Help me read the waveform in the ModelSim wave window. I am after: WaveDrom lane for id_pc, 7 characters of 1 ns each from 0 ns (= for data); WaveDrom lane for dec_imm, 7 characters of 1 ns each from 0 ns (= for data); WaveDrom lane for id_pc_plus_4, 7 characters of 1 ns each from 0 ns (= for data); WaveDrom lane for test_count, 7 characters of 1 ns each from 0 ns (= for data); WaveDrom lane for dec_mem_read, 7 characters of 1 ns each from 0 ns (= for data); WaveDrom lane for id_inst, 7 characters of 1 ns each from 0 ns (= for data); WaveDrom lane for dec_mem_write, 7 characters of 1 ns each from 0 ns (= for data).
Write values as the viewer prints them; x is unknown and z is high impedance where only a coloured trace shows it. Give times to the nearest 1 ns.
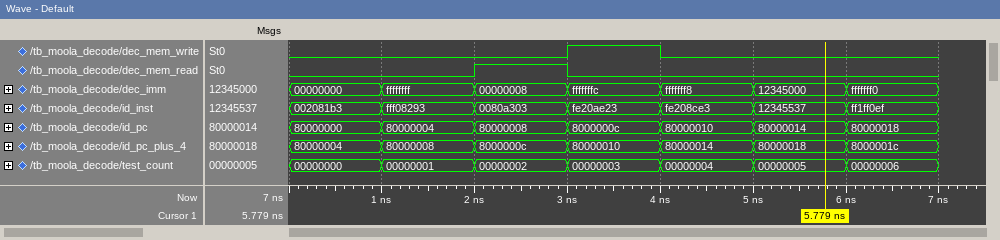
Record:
{name: 'id_pc', wave: '=======', data: '80000000 80000004 80000008 8000000c 80000010 80000014 80000018'}
{name: 'dec_imm', wave: '=======', data: '00000000 ffffffff 00000008 fffffffc fffffff8 12345000 fffffff0'}
{name: 'id_pc_plus_4', wave: '=======', data: '80000004 80000008 8000000c 80000010 80000014 80000018 8000001c'}
{name: 'test_count', wave: '=======', data: '00000000 00000001 00000002 00000003 00000004 00000005 00000006'}
{name: 'dec_mem_read', wave: '0.10...'}
{name: 'id_inst', wave: '=======', data: '002081b3 fff08293 0080a303 fe20ae23 fe208ce3 12345537 ff1ff0ef'}
{name: 'dec_mem_write', wave: '0..10..'}
